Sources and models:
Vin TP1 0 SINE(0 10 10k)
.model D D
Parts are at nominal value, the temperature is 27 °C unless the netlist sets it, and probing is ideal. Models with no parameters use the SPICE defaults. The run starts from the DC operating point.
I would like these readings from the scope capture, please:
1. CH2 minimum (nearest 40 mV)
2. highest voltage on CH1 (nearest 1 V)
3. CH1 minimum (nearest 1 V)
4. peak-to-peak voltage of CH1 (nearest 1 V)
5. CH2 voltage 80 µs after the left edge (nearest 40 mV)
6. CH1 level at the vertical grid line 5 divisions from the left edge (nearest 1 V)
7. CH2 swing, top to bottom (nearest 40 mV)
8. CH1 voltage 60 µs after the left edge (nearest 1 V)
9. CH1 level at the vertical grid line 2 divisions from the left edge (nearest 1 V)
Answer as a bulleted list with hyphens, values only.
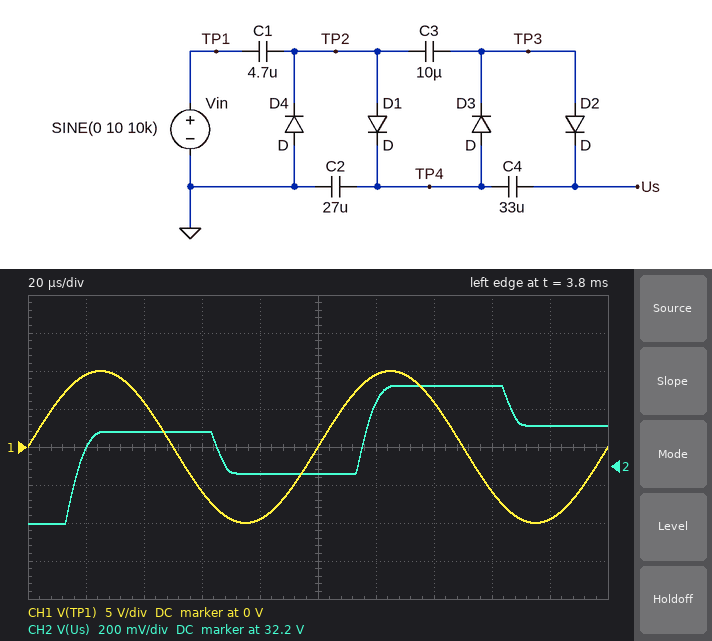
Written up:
- 31.88 V
- 10 V
- -10 V
- 20 V
- 32.16 V
- 0 V
- 720 mV
- -6 V
- 6 V
